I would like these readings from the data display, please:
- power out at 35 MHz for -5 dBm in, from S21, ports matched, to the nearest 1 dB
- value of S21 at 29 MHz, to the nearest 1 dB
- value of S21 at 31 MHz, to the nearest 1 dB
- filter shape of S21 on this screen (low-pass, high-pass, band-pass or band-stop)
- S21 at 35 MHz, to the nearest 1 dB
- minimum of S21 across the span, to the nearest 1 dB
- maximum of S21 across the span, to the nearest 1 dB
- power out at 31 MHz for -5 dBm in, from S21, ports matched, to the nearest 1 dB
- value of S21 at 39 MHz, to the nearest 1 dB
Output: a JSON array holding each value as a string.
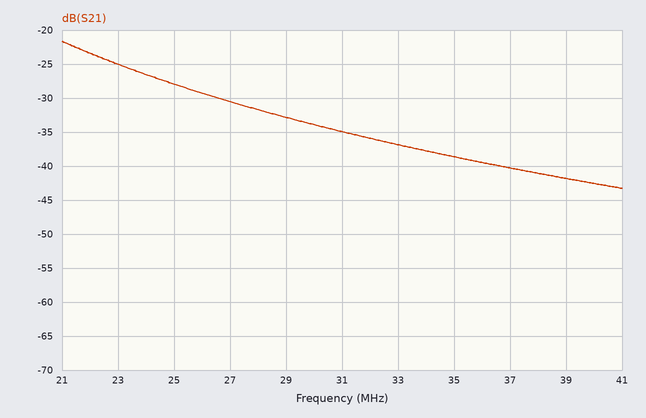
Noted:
["-44 dBm", "-33 dB", "-35 dB", "low-pass", "-39 dB", "-43 dB", "-22 dB", "-40 dBm", "-42 dB"]
